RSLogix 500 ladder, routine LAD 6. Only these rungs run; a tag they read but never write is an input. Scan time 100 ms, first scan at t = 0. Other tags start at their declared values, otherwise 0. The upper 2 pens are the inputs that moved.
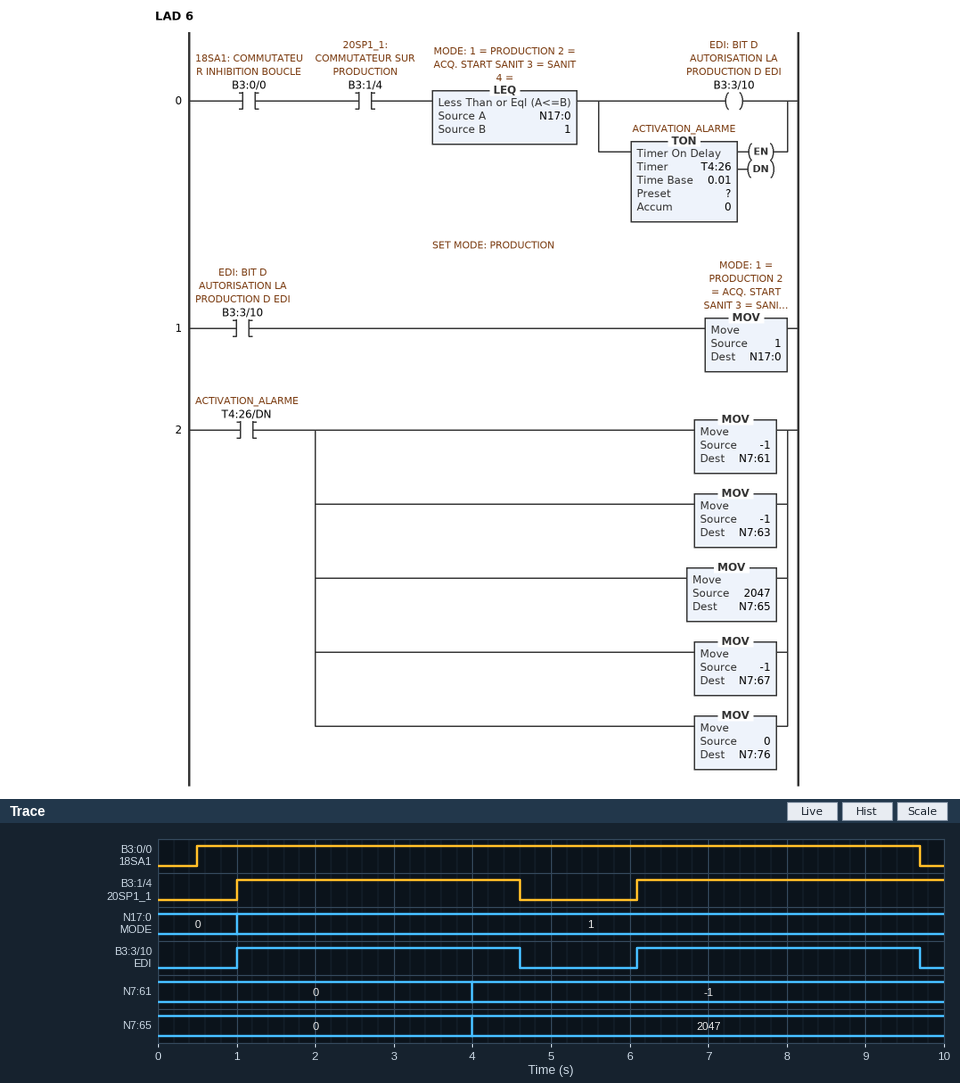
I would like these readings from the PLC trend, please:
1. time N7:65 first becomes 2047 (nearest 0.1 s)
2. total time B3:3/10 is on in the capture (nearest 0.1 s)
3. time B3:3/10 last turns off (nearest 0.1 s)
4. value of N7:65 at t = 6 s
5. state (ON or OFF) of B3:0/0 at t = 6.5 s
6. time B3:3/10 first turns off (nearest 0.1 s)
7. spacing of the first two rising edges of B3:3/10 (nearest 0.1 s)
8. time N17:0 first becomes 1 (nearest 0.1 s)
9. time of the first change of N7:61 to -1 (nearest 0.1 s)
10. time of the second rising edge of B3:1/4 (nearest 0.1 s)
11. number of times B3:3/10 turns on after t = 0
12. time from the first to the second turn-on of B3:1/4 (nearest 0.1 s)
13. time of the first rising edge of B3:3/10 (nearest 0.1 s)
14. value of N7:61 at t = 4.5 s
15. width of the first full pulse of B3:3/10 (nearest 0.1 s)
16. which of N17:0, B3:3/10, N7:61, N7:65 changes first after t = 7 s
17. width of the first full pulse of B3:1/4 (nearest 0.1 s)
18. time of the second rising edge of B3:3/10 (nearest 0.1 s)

4.0 s
7.2 s
9.7 s
2047
ON
4.6 s
5.1 s
1.0 s
4.0 s
6.1 s
2
5.1 s
1.0 s
-1
3.6 s
B3:3/10
3.6 s
6.1 s
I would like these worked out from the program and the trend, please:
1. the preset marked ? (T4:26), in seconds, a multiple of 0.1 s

3.0 s
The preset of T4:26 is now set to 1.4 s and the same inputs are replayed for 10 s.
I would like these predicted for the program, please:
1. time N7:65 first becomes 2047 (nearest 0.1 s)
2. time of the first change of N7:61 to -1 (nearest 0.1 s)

2.4 s
2.4 s
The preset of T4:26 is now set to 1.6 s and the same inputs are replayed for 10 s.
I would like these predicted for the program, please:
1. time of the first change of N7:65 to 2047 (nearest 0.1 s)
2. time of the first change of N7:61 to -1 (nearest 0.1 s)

2.6 s
2.6 s
